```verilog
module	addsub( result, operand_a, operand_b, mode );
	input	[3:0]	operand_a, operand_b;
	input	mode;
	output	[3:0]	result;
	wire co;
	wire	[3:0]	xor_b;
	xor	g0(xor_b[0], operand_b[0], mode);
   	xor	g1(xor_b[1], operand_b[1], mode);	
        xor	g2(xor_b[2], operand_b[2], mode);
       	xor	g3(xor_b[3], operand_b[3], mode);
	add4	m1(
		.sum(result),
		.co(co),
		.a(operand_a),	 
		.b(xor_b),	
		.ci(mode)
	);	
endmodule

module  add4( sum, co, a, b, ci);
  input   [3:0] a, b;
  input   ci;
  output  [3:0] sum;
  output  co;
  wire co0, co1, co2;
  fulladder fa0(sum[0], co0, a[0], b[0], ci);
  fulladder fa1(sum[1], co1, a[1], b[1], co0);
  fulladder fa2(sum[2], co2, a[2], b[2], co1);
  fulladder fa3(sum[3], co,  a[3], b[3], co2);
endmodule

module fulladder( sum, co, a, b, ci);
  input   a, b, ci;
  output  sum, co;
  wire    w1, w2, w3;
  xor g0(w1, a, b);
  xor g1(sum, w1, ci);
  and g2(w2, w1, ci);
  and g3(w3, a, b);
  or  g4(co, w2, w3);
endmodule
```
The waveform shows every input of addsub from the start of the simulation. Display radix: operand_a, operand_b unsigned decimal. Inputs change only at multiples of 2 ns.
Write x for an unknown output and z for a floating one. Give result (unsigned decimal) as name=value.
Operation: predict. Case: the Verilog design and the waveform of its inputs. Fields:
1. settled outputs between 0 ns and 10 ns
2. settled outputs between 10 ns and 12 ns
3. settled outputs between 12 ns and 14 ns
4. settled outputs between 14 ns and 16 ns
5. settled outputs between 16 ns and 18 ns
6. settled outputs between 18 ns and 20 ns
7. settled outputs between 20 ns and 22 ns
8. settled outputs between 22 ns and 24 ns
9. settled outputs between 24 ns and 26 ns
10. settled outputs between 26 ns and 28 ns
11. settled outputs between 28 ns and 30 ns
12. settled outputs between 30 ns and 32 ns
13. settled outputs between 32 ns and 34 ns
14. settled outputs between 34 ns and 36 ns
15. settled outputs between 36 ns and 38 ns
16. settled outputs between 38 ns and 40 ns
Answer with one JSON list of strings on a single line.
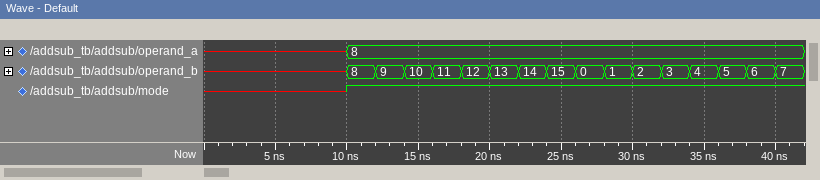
["result=x", "result=0", "result=15", "result=14", "result=13", "result=12", "result=11", "result=10", "result=9", "result=8", "result=7", "result=6", "result=5", "result=4", "result=3", "result=2"]
